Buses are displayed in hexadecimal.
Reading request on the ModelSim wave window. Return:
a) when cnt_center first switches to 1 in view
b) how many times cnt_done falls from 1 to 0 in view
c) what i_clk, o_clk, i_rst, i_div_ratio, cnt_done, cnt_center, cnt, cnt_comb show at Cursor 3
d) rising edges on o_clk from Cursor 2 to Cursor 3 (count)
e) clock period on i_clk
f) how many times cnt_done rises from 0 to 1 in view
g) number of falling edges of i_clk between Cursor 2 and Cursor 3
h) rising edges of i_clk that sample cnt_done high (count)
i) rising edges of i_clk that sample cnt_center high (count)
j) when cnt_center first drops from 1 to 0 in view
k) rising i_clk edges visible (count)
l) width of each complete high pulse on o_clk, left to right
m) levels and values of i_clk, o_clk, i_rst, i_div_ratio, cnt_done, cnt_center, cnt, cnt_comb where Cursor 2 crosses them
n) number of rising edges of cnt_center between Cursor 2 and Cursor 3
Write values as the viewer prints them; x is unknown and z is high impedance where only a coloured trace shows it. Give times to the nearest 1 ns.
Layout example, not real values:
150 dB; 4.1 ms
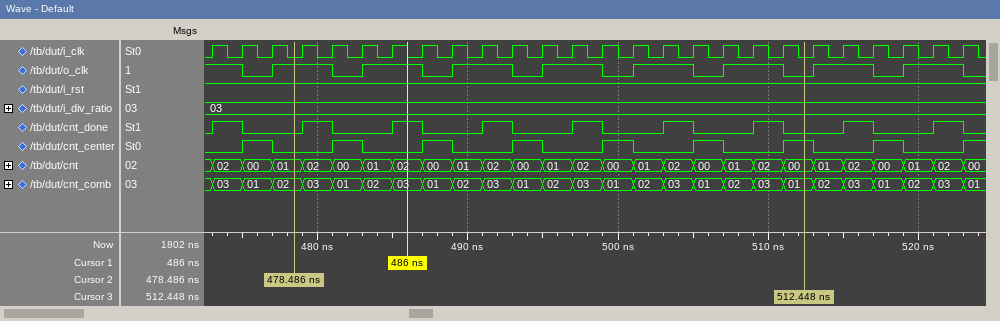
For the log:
475 ns; 9; i_clk=0, o_clk=0, i_rst=1, i_div_ratio=03, cnt_done=0, cnt_center=1, cnt=00, cnt_comb=01; 5; 2 ns; 9; 17; 9; 8; 477 ns; 26; 4 ns, 4 ns, 4 ns, 4 ns, 4 ns, 4 ns, 4 ns, 4 ns; i_clk=0, o_clk=1, i_rst=1, i_div_ratio=03, cnt_done=0, cnt_center=0, cnt=01, cnt_comb=02; 6
